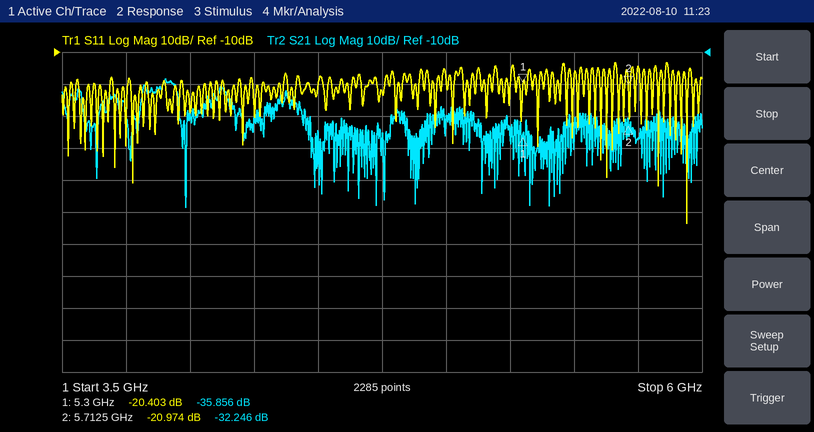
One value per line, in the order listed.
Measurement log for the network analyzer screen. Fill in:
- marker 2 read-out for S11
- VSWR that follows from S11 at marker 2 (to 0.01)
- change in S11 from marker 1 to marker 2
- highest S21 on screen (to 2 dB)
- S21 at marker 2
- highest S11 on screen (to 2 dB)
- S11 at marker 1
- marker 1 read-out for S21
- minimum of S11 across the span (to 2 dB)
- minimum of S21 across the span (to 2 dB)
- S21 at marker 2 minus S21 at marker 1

-20.974 dB
1.20
-0.571 dB
-18 dB
-32.246 dB
-14 dB
-20.403 dB
-35.856 dB
-64 dB
-58 dB
3.610 dB
